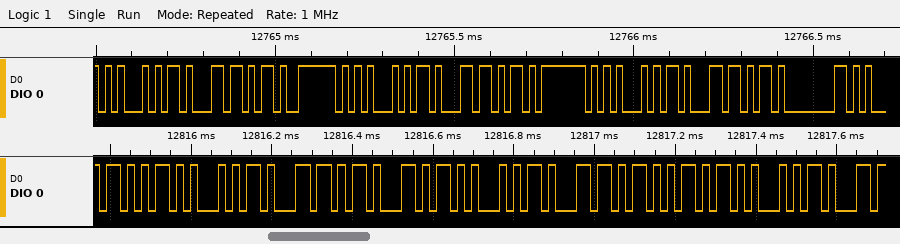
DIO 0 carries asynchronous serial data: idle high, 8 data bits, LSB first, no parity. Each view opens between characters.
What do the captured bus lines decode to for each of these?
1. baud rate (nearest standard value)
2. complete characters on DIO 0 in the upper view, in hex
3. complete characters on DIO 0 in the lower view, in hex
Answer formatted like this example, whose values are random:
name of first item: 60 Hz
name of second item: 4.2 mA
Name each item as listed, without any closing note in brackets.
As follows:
baud rate: 57600 baud
complete characters on DIO 0 in the upper view, in hex: 45, 8B, 6B, 7E, 45, 8B, 6B, 7F, 45, 8B, 6B, 80
complete characters on DIO 0 in the lower view, in hex: AB, 45, 8B, 6B, AC, 45, 8B, 6B, AD, 45, 8B
